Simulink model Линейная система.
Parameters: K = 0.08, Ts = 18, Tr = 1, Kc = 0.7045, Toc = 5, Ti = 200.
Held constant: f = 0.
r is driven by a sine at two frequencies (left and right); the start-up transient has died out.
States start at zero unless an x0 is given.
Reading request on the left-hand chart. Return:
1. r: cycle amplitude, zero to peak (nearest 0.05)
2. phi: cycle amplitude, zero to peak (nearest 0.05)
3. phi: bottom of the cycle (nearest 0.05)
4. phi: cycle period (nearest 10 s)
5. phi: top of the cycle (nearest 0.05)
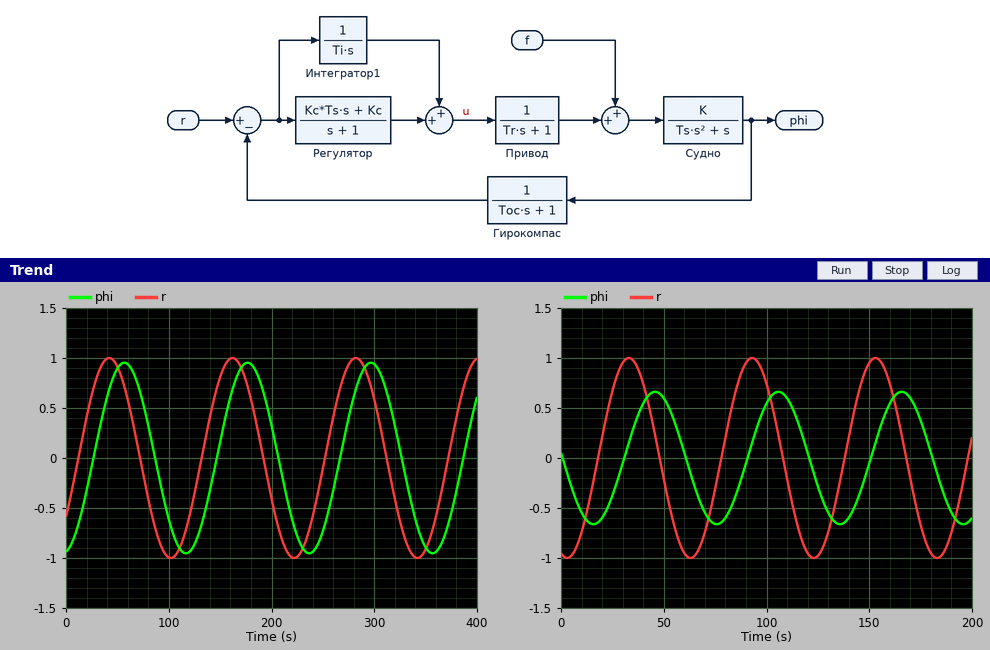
1.00
0.95
-0.95
120 s
0.95
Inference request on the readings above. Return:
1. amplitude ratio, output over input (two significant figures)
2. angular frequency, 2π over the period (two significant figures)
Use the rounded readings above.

0.95
0.052 rad/s
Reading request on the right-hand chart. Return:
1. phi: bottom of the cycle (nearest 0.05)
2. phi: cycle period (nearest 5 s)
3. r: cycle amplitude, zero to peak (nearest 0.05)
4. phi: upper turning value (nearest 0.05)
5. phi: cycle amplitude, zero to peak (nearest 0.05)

-0.65
60 s
1.00
0.65
0.65
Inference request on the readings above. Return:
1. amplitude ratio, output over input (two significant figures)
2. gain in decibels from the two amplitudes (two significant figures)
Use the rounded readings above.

0.65
-3.7 dB
